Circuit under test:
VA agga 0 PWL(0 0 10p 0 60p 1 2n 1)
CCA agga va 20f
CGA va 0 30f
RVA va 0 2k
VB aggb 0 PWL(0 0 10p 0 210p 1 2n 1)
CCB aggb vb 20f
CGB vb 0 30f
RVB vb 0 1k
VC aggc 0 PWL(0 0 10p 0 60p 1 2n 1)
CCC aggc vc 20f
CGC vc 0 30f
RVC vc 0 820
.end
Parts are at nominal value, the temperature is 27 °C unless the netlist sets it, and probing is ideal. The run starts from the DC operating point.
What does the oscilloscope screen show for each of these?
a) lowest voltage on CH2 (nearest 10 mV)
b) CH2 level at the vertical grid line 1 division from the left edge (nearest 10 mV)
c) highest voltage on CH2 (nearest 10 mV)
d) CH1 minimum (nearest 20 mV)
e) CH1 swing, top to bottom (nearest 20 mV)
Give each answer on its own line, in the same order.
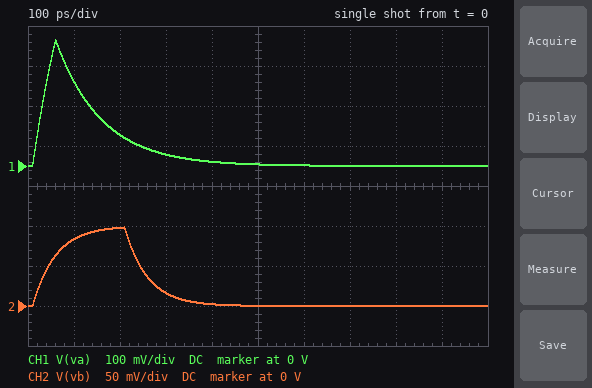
0 V
80 mV
100 mV
0 V
320 mV
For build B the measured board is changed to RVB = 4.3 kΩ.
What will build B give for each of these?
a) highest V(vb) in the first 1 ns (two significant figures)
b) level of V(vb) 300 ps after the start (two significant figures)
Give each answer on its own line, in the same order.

260 mV
170 mV
